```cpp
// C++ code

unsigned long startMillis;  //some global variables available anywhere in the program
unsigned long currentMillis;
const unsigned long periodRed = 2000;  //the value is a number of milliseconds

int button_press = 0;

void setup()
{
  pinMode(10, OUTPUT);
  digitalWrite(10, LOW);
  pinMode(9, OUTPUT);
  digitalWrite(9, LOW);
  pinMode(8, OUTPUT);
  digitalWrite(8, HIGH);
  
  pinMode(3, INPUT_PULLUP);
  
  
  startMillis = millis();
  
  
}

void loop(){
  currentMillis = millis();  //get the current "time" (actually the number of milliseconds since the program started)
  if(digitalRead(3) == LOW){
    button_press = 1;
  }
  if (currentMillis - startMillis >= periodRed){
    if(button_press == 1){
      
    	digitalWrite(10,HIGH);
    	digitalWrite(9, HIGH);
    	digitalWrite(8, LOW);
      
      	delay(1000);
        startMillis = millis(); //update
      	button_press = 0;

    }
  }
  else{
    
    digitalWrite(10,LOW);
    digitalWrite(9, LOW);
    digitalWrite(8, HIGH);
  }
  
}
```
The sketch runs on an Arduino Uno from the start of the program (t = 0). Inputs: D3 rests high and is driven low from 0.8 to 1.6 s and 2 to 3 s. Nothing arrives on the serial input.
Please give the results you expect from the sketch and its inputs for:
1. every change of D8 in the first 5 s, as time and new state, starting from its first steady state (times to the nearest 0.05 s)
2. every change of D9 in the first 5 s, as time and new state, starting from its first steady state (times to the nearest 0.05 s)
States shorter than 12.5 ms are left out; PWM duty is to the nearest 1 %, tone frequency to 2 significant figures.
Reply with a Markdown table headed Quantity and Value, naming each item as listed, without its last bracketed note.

| Quantity | Value |
|---|---|
| every change of D8 in the first 5 s, as time and new state, starting from its first steady state | 0 s high; 2 s low; 3 s high |
| every change of D9 in the first 5 s, as time and new state, starting from its first steady state | 0 s low; 2 s high; 3 s low |
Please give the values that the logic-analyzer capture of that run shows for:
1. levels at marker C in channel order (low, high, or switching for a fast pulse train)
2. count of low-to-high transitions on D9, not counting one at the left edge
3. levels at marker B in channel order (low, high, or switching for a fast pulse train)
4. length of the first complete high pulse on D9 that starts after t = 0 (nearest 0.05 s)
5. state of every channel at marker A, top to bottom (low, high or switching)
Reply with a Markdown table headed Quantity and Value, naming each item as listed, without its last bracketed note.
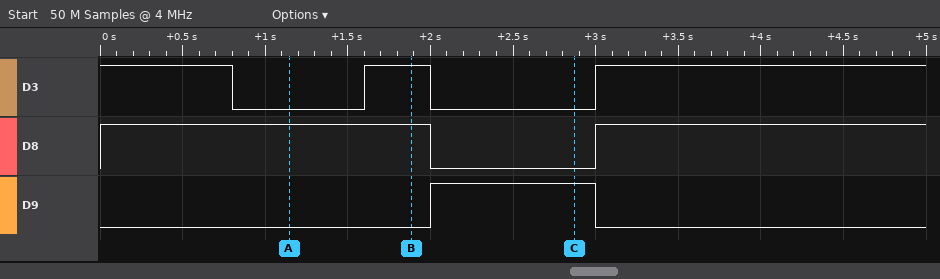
| Quantity | Value |
|---|---|
| levels at marker C in channel order | D3 low, D8 low, D9 high |
| count of low-to-high transitions on D9, not counting one at the left edge | 1 |
| levels at marker B in channel order | D3 high, D8 high, D9 low |
| length of the first complete high pulse on D9 that starts after t = 0 | 1.00 s |
| state of every channel at marker A, top to bottom | D3 low, D8 high, D9 low |
